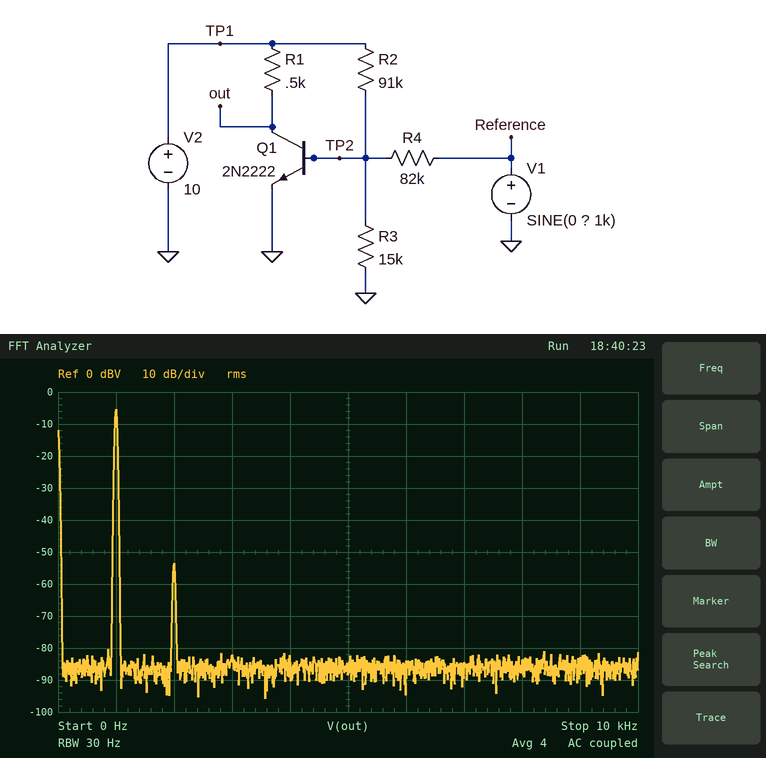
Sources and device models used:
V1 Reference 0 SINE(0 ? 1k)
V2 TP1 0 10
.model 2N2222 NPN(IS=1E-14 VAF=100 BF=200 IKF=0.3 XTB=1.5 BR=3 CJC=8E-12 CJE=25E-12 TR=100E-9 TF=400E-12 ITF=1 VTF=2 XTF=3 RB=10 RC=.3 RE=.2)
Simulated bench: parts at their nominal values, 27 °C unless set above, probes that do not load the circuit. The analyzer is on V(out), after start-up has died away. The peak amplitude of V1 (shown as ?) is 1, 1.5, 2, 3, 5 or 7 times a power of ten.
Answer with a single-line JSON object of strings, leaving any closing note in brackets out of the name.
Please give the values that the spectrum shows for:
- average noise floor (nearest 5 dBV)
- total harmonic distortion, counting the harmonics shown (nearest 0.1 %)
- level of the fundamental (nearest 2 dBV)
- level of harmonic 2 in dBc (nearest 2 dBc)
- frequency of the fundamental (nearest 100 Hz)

{"average noise floor": "-85 dBV", "total harmonic distortion, counting the harmonics shown": "0.4 %", "level of the fundamental": "-6 dBV", "level of harmonic 2 in dBc": "-48 dBc", "frequency of the fundamental": "1.0 kHz"}
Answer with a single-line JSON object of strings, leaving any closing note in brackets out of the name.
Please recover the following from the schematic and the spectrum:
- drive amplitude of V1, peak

{"drive amplitude of V1, peak": "700 mV"}
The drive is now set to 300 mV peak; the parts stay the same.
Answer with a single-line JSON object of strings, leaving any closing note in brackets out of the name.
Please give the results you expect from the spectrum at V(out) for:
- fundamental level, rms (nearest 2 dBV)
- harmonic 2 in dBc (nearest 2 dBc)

{"fundamental level, rms": "-12 dBV", "harmonic 2 in dBc": "-56 dBc"}
